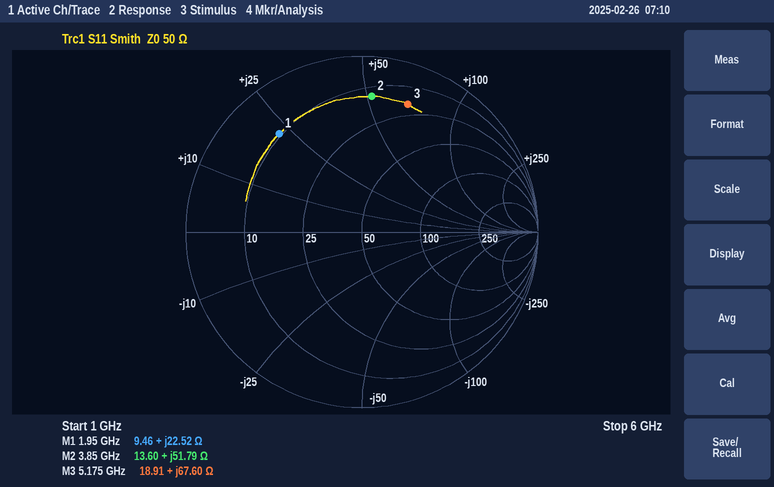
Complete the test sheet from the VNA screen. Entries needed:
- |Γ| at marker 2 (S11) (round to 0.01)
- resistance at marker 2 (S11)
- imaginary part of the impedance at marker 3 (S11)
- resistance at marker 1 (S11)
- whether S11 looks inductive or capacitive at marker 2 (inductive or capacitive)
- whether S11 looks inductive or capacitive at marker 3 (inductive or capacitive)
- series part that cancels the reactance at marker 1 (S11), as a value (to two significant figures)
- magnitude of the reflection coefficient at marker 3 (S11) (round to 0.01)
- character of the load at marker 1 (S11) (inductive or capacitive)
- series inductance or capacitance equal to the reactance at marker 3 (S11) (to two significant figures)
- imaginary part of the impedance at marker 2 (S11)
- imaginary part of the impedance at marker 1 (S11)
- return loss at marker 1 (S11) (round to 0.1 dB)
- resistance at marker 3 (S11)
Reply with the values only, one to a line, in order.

0.77
13.60 Ω
+67.60 Ω
9.46 Ω
inductive
inductive
3.6 pF
0.77
inductive
2.1 nH
+51.79 Ω
+22.52 Ω
2.7 dB
18.91 Ω
